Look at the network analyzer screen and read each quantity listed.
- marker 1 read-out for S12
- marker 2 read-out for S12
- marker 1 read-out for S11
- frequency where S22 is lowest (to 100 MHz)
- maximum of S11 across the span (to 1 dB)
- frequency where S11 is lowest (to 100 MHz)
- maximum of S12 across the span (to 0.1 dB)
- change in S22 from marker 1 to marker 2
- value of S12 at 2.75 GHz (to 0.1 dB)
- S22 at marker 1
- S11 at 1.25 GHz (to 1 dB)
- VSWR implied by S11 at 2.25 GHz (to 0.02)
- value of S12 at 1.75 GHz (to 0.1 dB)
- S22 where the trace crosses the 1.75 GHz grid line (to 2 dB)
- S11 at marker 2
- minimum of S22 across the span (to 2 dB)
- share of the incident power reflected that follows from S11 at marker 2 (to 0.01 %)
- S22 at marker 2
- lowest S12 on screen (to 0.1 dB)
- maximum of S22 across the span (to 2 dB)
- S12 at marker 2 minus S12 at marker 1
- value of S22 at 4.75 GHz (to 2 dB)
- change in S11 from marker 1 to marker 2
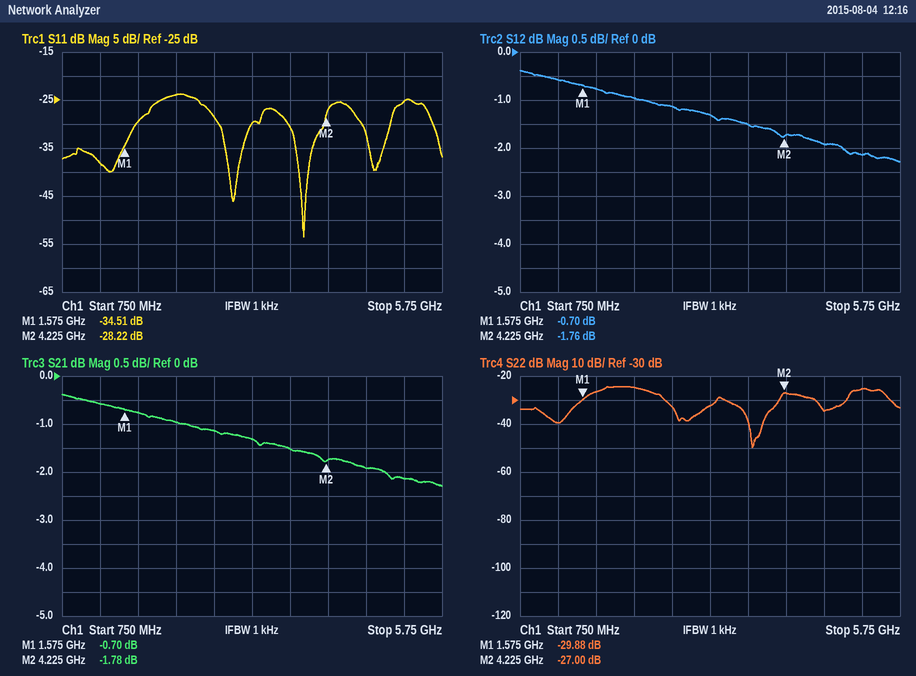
-0.70 dB
-1.76 dB
-34.51 dB
3.8 GHz
-24 dB
3.9 GHz
-0.4 dB
2.88 dB
-1.1 dB
-29.88 dB
-38 dB
1.14
-0.8 dB
-26 dB
-28.22 dB
-50 dB
0.15 %
-27.00 dB
-2.3 dB
-24 dB
-1.06 dB
-34 dB
6.29 dB
